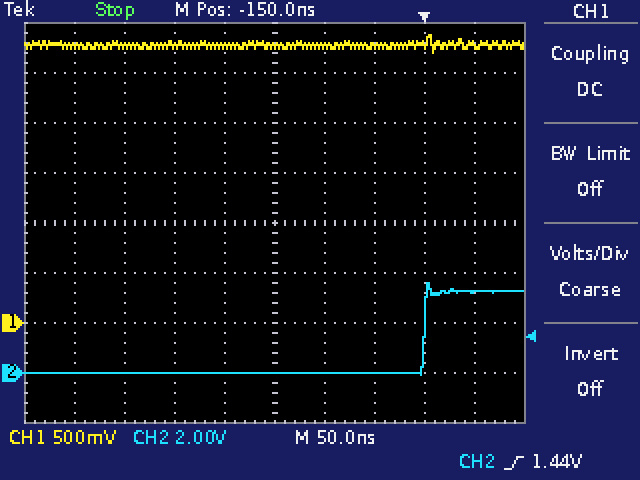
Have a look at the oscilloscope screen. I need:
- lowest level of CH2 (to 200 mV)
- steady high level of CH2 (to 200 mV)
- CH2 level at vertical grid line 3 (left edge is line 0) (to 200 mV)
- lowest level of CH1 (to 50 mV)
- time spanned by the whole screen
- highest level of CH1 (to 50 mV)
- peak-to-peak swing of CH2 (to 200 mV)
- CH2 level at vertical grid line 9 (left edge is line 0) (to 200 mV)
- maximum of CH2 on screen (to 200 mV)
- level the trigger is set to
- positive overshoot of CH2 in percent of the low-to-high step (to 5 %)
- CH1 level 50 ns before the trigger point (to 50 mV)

0.0 V
3.2 V
0.0 V
2.70 V
500 ns
2.90 V
3.6 V
3.2 V
3.6 V
1.44 V
10 %
2.75 V
